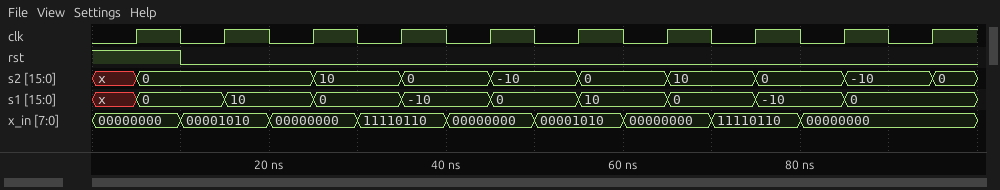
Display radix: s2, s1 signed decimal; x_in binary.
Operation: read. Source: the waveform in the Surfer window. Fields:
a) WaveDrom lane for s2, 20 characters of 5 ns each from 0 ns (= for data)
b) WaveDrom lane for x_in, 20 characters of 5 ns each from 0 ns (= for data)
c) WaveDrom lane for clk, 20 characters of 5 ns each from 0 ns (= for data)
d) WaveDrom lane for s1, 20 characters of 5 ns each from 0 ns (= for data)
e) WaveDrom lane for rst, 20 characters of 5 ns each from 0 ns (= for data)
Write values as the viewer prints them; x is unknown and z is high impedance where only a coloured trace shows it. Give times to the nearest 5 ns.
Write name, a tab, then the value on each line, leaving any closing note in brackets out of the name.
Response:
WaveDrom lane for s2, 20 characters of 5 ns each from 0 ns	{name: 's2', wave: 'x=...=.=.=.=.=.=.=.=', data: '0 10 0 -10 0 10 0 -10 0'}
WaveDrom lane for x_in, 20 characters of 5 ns each from 0 ns	{name: 'x_in', wave: '=.=.=.=.=.=.=.=.=...', data: '00000000 00001010 00000000 11110110 00000000 00001010 00000000 11110110 00000000'}
WaveDrom lane for clk, 20 characters of 5 ns each from 0 ns	{name: 'clk', wave: '01010101010101010101'}
WaveDrom lane for s1, 20 characters of 5 ns each from 0 ns	{name: 's1', wave: 'x=.=.=.=.=.=.=.=.=..', data: '0 10 0 -10 0 10 0 -10 0'}
WaveDrom lane for rst, 20 characters of 5 ns each from 0 ns	{name: 'rst', wave: '1.0.................'}
